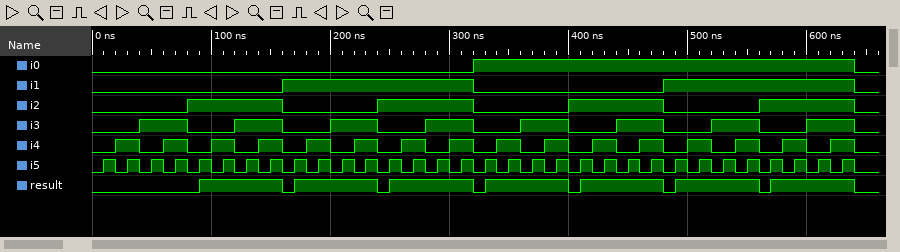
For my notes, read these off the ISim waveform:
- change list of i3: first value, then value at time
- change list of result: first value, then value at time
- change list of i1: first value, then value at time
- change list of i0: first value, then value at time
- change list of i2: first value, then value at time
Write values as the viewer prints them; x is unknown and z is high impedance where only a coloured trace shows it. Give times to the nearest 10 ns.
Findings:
0, 1 at 40 ns, 0 at 80 ns, 1 at 120 ns, 0 at 160 ns, 1 at 200 ns, 0 at 240 ns, 1 at 280 ns, 0 at 320 ns, 1 at 360 ns, 0 at 400 ns, 1 at 440 ns, 0 at 480 ns, 1 at 520 ns, 0 at 560 ns, 1 at 600 ns, 0 at 640 ns
0, 1 at 90 ns, 0 at 160 ns, 1 at 170 ns, 0 at 240 ns, 1 at 250 ns, 0 at 320 ns, 1 at 330 ns, 0 at 400 ns, 1 at 410 ns, 0 at 480 ns, 1 at 490 ns, 0 at 560 ns, 1 at 570 ns, 0 at 640 ns
0, 1 at 160 ns, 0 at 320 ns, 1 at 480 ns, 0 at 640 ns
0, 1 at 320 ns, 0 at 640 ns
0, 1 at 80 ns, 0 at 160 ns, 1 at 240 ns, 0 at 320 ns, 1 at 400 ns, 0 at 480 ns, 1 at 560 ns, 0 at 640 ns
